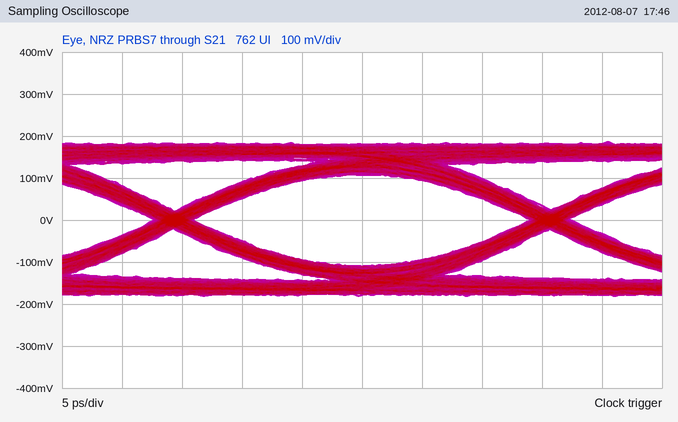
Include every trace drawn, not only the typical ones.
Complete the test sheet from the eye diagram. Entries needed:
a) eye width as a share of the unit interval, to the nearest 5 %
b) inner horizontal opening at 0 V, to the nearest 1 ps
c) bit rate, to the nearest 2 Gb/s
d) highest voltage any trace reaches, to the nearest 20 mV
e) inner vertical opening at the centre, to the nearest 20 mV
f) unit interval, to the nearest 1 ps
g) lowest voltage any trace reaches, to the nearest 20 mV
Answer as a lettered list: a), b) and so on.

a) 90 %
b) 28 ps
c) 32 Gb/s
d) 180 mV
e) 220 mV
f) 31 ps
g) -180 mV
